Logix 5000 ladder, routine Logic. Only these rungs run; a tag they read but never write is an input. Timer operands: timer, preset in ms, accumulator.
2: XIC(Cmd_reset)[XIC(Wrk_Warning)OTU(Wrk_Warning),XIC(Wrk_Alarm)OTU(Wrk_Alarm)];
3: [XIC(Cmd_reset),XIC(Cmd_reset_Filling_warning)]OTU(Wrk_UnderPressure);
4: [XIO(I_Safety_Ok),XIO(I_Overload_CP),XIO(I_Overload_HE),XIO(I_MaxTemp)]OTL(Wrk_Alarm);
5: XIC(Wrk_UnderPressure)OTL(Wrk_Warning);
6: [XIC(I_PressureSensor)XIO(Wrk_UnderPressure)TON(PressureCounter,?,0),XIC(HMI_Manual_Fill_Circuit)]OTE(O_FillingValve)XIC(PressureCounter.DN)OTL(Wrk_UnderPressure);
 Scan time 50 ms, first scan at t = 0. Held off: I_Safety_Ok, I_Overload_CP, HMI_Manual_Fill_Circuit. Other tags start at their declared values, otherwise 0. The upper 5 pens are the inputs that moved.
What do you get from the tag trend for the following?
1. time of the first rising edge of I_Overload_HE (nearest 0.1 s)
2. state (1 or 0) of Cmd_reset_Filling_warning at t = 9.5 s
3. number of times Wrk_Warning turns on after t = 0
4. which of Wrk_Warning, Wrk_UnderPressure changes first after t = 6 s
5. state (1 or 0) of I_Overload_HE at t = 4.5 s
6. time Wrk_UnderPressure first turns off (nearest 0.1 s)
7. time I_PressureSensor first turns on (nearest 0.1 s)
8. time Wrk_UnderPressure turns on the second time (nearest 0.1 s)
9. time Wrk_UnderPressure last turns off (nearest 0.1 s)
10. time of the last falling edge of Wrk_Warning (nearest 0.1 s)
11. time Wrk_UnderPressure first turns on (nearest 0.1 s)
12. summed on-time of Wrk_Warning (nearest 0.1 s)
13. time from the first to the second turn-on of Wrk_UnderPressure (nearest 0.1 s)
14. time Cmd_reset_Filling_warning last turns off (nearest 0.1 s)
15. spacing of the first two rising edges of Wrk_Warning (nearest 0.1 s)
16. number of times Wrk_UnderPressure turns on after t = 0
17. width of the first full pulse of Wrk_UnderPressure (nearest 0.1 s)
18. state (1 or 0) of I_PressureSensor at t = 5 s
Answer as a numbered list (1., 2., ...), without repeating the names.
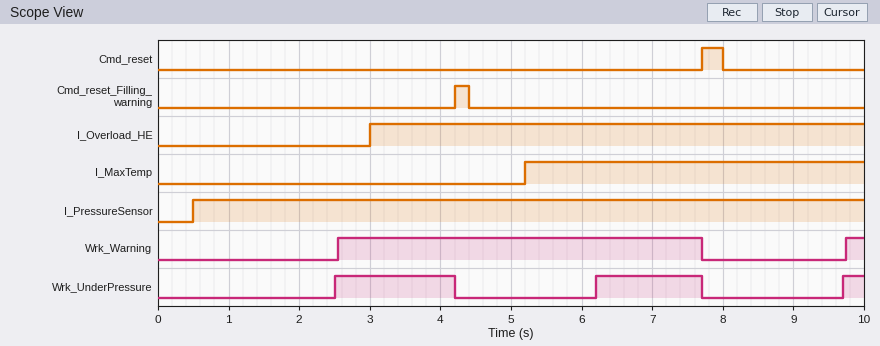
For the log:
1. 3.0 s
2. 0
3. 2
4. Wrk_UnderPressure
5. 1
6. 4.2 s
7. 0.5 s
8. 6.2 s
9. 7.7 s
10. 7.7 s
11. 2.5 s
12. 5.4 s
13. 3.7 s
14. 4.4 s
15. 7.2 s
16. 3
17. 1.7 s
18. 1
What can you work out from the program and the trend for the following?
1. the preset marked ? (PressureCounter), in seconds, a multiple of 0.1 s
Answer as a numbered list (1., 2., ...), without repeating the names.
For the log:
1. 2.0 s
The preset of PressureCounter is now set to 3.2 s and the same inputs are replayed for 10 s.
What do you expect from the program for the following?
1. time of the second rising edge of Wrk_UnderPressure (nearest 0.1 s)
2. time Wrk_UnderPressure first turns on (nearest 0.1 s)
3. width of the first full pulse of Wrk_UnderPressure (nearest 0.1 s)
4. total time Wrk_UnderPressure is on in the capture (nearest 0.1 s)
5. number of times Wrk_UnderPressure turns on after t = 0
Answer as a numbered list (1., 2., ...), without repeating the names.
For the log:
1. 7.4 s
2. 3.7 s
3. 0.5 s
4. 0.8 s
5. 2
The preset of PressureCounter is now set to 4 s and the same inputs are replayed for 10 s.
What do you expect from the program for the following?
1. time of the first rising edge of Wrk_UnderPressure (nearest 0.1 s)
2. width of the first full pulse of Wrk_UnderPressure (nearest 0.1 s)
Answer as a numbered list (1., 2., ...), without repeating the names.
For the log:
1. 4.5 s
2. 3.2 s
